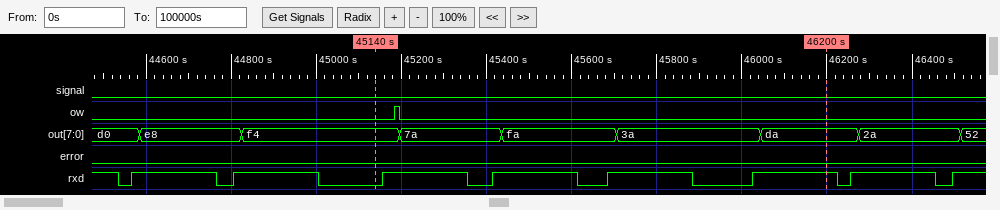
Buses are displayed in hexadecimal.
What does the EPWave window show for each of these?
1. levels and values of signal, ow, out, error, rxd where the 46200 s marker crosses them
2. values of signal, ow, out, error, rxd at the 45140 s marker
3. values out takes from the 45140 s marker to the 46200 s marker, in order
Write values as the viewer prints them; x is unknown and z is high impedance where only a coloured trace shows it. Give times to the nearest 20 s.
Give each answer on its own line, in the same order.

signal=0, ow=0, out=da, error=0, rxd=1
signal=0, ow=0, out=f4, error=0, rxd=0
f4, 7a, fa, 3a, da
